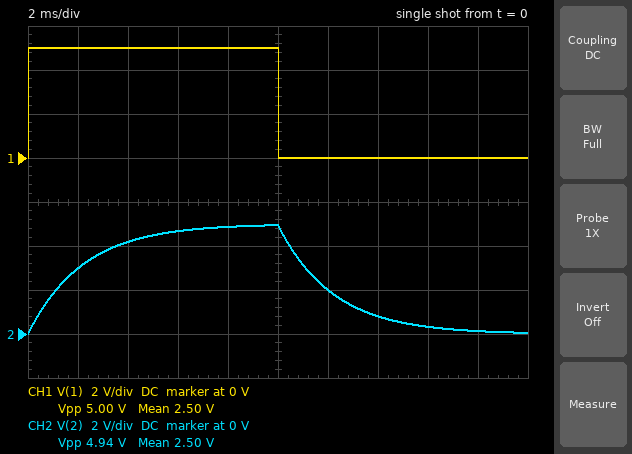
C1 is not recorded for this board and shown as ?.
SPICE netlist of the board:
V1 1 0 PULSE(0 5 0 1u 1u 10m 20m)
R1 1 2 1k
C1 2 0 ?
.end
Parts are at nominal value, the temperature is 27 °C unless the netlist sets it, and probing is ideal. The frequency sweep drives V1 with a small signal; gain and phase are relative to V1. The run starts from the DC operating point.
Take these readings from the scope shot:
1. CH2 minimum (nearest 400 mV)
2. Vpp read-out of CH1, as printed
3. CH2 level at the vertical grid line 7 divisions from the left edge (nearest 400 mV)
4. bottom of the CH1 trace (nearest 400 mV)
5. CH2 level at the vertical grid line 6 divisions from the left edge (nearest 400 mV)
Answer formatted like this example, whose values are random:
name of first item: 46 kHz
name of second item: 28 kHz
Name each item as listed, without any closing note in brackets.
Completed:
CH2 minimum: 0 V
Vpp read-out of CH1, as printed: 5.00 V
CH2 level at the vertical grid line 7 divisions from the left edge: 800 mV
bottom of the CH1 trace: 0 V
CH2 level at the vertical grid line 6 divisions from the left edge: 2.0 V
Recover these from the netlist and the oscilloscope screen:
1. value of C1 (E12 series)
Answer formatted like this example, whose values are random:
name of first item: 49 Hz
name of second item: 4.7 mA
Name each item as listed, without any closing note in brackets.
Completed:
value of C1: 2.2 µF
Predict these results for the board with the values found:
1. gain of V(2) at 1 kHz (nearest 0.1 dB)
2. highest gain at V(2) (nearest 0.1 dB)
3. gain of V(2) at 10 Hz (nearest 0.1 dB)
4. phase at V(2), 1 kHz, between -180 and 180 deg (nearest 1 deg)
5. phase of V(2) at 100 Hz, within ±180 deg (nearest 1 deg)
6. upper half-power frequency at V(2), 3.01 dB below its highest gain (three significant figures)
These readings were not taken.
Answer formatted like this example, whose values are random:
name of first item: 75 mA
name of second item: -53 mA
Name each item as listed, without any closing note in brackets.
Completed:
gain of V(2) at 1 kHz: -22.8 dB
highest gain at V(2): 0 dB
gain of V(2) at 10 Hz: -0.1 dB
phase at V(2), 1 kHz, between -180 and 180 deg: -86 deg
phase of V(2) at 100 Hz, within ±180 deg: -54 deg
upper half-power frequency at V(2), 3.01 dB below its highest gain: 72.3 Hz
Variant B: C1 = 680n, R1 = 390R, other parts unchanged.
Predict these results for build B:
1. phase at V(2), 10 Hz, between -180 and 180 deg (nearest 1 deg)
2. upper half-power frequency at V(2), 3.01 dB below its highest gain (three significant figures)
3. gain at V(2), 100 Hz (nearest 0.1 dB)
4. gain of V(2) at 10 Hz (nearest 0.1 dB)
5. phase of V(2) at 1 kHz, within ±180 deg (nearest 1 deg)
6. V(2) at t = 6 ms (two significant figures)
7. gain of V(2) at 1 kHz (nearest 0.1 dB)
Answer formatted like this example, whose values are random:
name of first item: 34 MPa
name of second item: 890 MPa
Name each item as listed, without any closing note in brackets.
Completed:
phase at V(2), 10 Hz, between -180 and 180 deg: -1 deg
upper half-power frequency at V(2), 3.01 dB below its highest gain: 600 Hz
gain at V(2), 100 Hz: -0.1 dB
gain of V(2) at 10 Hz: 0 dB
phase of V(2) at 1 kHz, within ±180 deg: -59 deg
V(2) at t = 6 ms: 5.0 V
gain of V(2) at 1 kHz: -5.8 dB
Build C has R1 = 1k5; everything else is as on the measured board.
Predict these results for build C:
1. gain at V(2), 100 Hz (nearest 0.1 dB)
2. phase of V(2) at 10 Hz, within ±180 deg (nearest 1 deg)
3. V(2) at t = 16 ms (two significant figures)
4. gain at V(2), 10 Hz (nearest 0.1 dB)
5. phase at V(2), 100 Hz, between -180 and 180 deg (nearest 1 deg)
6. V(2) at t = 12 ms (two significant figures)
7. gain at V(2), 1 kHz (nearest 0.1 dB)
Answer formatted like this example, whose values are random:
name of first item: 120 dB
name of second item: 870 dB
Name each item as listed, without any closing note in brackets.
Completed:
gain at V(2), 100 Hz: -7.2 dB
phase of V(2) at 10 Hz, within ±180 deg: -12 deg
V(2) at t = 16 ms: 770 mV
gain at V(2), 10 Hz: -0.2 dB
phase at V(2), 100 Hz, between -180 and 180 deg: -64 deg
V(2) at t = 12 ms: 2.6 V
gain at V(2), 1 kHz: -26.3 dB
